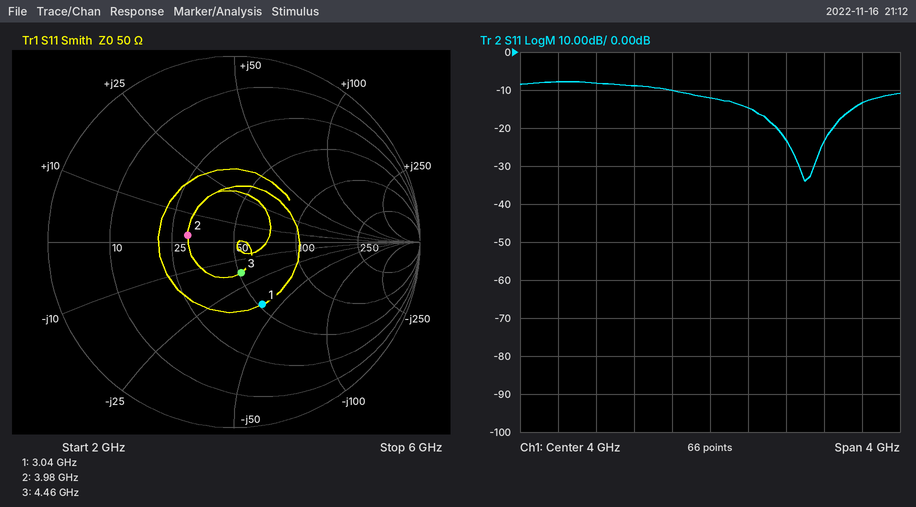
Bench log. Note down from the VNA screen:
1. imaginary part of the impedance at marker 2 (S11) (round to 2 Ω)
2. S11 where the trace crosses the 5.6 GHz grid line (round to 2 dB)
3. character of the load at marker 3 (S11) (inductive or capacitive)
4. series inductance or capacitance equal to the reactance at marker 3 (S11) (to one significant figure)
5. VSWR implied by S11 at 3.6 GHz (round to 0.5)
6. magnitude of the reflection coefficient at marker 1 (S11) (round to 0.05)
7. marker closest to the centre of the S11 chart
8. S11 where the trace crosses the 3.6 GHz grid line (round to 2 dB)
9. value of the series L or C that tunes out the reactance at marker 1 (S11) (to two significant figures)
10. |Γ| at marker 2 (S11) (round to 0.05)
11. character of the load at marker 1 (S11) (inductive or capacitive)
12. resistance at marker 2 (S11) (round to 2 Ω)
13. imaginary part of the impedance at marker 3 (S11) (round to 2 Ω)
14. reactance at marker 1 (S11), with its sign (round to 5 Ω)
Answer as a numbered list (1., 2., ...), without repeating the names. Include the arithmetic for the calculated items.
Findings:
1. +2 Ω
2. -14 dB
3. capacitive
4. C = 1/(2π × 4.46 GHz × 18 Ω) ≈ 2 pF
5. |Γ| = 10^(-10/20) = 0.3162; VSWR = (1 + 0.3162)/(1 − 0.3162) ≈ 1.92, so 2.0 to the nearest 0.5
6. 0.35
7. marker 3
8. -10 dB
9. L = 40 Ω/(2π × 3.04 GHz) ≈ 2.1 nH
10. 0.25
11. capacitive
12. 30 Ω
13. -18 Ω
14. -40 Ω
